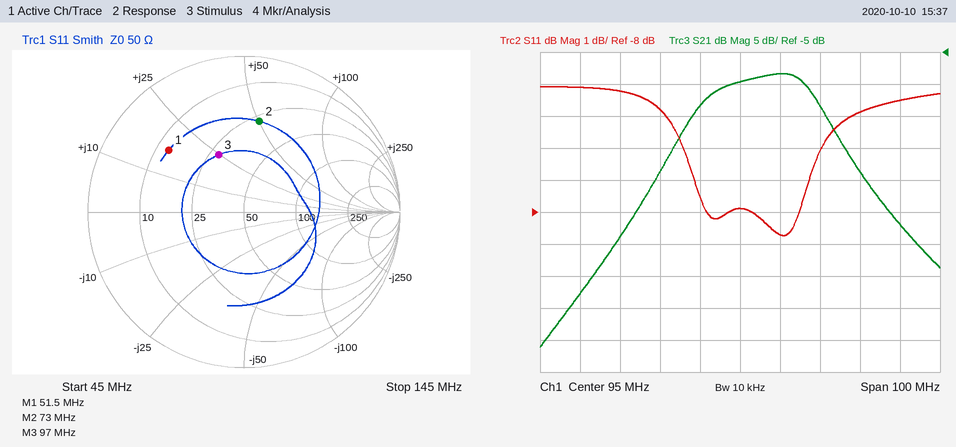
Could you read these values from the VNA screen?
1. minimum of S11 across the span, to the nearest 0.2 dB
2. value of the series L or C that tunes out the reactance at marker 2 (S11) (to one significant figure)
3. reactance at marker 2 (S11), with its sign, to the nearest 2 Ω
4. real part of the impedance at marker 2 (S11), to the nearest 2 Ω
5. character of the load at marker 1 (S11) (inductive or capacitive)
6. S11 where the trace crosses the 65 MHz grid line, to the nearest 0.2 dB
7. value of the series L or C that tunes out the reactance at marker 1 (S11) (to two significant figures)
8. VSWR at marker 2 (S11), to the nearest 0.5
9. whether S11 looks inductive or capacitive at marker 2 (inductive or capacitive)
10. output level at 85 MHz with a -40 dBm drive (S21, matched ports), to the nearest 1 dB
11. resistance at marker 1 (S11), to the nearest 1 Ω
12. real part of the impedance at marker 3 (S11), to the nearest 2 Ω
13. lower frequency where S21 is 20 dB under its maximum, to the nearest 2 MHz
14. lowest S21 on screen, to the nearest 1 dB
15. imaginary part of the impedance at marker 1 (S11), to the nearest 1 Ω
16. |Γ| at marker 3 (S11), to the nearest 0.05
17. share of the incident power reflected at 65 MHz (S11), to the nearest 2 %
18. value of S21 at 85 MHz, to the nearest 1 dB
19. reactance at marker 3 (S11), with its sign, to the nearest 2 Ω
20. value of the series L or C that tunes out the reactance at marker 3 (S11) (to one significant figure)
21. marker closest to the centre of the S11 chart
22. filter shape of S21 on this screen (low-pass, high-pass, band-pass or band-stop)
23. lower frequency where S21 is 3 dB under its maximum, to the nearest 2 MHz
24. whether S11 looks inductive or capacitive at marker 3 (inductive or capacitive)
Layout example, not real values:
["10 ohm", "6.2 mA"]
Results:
["-8.8 dB", "40 pF", "+50 Ω", "28 Ω", "inductive", "-4.2 dB", "180 pF", "4.0", "inductive", "-53 dBm", "13 Ω", "28 Ω", "70 MHz", "-51 dB", "+17 Ω", "0.40", "38 %", "-13 dB", "+24 Ω", "70 pF", "marker 3", "band-pass", "88 MHz", "inductive"]
